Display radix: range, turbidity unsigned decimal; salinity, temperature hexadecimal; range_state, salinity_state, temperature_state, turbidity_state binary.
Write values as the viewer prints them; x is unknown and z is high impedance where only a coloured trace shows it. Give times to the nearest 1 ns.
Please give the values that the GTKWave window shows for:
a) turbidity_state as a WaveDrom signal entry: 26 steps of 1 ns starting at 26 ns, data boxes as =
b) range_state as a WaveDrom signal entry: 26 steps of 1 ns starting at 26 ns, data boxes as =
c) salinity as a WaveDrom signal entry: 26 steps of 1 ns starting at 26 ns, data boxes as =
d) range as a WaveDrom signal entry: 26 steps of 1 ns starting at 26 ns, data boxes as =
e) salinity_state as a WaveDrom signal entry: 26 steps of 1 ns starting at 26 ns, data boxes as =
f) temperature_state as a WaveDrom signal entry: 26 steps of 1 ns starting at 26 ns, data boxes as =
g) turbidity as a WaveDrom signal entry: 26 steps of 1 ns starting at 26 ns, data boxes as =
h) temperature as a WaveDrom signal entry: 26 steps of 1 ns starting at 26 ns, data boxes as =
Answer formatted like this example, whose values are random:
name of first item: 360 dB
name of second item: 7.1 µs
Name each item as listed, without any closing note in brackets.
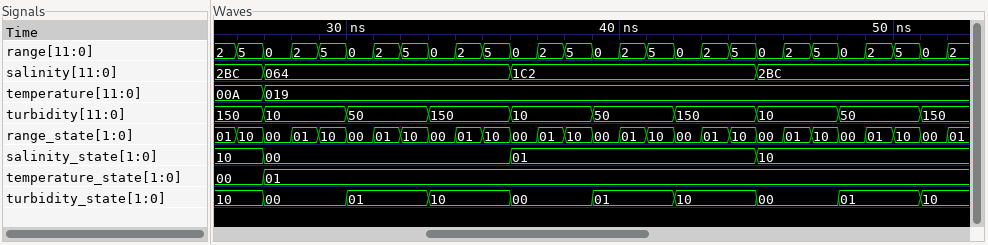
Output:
turbidity_state as a WaveDrom signal entry: 26 steps of 1 ns starting at 26 ns, data boxes as =: {name: 'turbidity_state', wave: '==..=..=..=..=..=..=..=..=', data: '10 00 01 10 00 01 10 00 01 10'}
range_state as a WaveDrom signal entry: 26 steps of 1 ns starting at 26 ns, data boxes as =: {name: 'range_state', wave: '==========================', data: '10 00 01 10 00 01 10 00 01 10 00 01 10 00 01 10 00 01 10 00 01 10 00 01 10 00'}
salinity as a WaveDrom signal entry: 26 steps of 1 ns starting at 26 ns, data boxes as =: {name: 'salinity', wave: '==........=........=......', data: '2BC 064 1C2 2BC'}
range as a WaveDrom signal entry: 26 steps of 1 ns starting at 26 ns, data boxes as =: {name: 'range', wave: '==========================', data: '5 0 2 5 0 2 5 0 2 5 0 2 5 0 2 5 0 2 5 0 2 5 0 2 5 0'}
salinity_state as a WaveDrom signal entry: 26 steps of 1 ns starting at 26 ns, data boxes as =: {name: 'salinity_state', wave: '==........=........=......', data: '10 00 01 10'}
temperature_state as a WaveDrom signal entry: 26 steps of 1 ns starting at 26 ns, data boxes as =: {name: 'temperature_state', wave: '==........................', data: '00 01'}
turbidity as a WaveDrom signal entry: 26 steps of 1 ns starting at 26 ns, data boxes as =: {name: 'turbidity', wave: '==..=..=..=..=..=..=..=..=', data: '150 10 50 150 10 50 150 10 50 150'}
temperature as a WaveDrom signal entry: 26 steps of 1 ns starting at 26 ns, data boxes as =: {name: 'temperature', wave: '==........................', data: '00A 019'}
